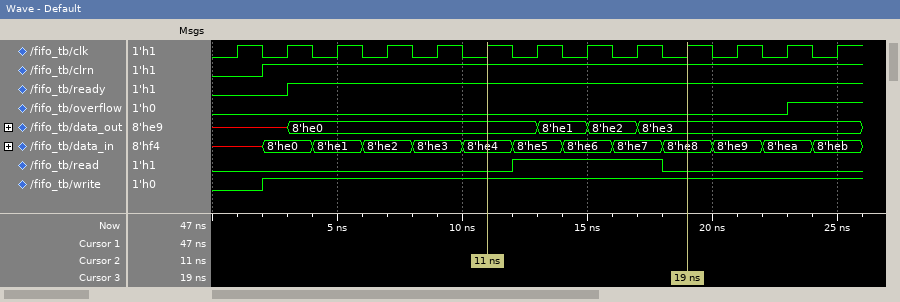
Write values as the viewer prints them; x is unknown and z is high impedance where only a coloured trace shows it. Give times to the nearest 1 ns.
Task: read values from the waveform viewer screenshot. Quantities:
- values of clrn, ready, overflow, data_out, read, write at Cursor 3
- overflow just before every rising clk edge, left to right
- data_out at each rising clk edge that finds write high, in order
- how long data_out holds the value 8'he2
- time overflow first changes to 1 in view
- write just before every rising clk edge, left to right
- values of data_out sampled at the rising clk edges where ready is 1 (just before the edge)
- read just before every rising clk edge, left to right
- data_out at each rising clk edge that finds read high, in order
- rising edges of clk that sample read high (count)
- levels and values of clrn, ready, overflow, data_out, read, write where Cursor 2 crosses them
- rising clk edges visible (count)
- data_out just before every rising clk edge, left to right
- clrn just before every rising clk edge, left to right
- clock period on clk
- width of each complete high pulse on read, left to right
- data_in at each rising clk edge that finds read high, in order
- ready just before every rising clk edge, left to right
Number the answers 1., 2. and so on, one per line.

1. clrn=1, ready=1, overflow=0, data_out=8'he3, read=0, write=1
2. 0 0 0 0 0 0 0 0 0 0 0 0 1
3. x, 8'he0, 8'he0, 8'he0, 8'he0, 8'he0, 8'he1, 8'he2, 8'he3, 8'he3, 8'he3, 8'he3
4. 2 ns
5. 23 ns
6. 0 1 1 1 1 1 1 1 1 1 1 1 1
7. 8'he0, 8'he0, 8'he0, 8'he0, 8'he0, 8'he1, 8'he2, 8'he3, 8'he3, 8'he3, 8'he3
8. 0 0 0 0 0 0 1 1 1 0 0 0 0
9. 8'he0, 8'he1, 8'he2
10. 3
11. clrn=1, ready=1, overflow=0, data_out=8'he0, read=0, write=1
12. 13
13. x, x, 8'he0, 8'he0, 8'he0, 8'he0, 8'he0, 8'he1, 8'he2, 8'he3, 8'he3, 8'he3, 8'he3
14. 0 1 1 1 1 1 1 1 1 1 1 1 1
15. 2 ns
16. 6 ns
17. 8'he5, 8'he6, 8'he7
18. 0 0 1 1 1 1 1 1 1 1 1 1 1
